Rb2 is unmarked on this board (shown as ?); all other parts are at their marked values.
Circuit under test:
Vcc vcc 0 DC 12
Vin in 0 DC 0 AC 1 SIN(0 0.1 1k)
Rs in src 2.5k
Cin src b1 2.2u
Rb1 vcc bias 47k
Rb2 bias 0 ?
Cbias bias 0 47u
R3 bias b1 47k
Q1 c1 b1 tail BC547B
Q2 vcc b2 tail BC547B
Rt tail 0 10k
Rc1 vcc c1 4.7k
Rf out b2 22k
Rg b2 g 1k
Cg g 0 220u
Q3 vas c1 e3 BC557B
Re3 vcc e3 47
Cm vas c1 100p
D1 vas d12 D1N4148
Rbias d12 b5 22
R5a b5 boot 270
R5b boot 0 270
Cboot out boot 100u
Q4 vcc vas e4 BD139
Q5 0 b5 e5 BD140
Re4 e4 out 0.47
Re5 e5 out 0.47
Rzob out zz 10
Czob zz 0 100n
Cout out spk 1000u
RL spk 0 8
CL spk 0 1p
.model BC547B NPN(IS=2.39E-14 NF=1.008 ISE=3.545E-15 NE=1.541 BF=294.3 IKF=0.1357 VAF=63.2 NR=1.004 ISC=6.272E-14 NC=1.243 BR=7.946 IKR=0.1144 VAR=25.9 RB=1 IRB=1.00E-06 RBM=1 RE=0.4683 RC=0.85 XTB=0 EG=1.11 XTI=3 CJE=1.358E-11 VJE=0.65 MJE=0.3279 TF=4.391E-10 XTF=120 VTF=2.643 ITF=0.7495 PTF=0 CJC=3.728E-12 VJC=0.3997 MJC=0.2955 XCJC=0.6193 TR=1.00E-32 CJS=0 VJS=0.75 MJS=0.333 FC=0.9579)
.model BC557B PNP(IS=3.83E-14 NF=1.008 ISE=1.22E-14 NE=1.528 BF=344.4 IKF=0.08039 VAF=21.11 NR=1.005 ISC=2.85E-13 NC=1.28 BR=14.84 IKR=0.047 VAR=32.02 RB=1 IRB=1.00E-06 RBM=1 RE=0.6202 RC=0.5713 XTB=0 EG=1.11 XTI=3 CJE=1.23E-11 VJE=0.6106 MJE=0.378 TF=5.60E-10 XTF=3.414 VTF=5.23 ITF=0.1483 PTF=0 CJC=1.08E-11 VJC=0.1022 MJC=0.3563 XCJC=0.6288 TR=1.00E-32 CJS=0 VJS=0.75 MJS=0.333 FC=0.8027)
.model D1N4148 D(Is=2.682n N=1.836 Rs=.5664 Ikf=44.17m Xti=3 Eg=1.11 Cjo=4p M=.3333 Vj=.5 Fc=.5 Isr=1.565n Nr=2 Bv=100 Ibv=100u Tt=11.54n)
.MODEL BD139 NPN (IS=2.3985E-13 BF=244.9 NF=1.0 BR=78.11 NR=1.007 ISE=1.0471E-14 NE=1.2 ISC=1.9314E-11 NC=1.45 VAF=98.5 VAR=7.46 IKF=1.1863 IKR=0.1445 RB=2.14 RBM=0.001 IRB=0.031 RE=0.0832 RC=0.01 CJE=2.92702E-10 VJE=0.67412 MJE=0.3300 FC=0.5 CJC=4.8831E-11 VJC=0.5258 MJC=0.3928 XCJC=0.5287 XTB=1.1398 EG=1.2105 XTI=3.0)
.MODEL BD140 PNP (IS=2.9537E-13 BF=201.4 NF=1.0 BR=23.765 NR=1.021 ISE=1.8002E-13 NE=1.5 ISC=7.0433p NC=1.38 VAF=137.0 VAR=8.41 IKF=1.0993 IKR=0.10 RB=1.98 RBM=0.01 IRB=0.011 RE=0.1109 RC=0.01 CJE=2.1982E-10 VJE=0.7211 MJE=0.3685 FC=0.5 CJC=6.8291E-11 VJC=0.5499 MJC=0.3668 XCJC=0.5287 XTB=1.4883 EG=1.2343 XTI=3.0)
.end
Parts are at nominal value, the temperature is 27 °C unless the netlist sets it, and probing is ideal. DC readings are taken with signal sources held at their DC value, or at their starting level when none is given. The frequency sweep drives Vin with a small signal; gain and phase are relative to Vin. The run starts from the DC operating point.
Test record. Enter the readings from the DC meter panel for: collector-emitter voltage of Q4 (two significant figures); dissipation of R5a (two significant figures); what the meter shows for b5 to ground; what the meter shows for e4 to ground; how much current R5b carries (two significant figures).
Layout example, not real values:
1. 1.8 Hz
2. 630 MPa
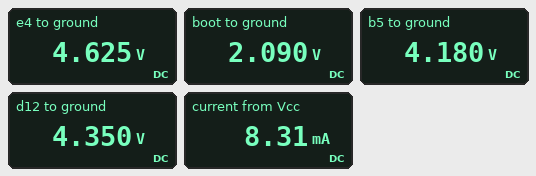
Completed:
1. 7.4 V
2. 16 mW
3. 4.180 V
4. 4.625 V
5. 7.7 mA
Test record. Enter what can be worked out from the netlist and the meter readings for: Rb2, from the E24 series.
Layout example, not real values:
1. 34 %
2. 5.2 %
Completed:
1. 30 kΩ
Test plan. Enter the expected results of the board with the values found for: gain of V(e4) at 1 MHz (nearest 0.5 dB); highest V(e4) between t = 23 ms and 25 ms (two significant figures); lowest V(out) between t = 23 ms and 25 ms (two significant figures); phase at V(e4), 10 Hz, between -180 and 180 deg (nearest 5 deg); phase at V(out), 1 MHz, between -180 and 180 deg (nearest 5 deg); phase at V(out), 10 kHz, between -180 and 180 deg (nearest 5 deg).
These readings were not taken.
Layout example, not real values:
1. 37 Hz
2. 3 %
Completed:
1. -20.5 dB
2. 6.7 V
3. 2.7 V
4. -20 deg
5. -80 deg
6. -10 deg
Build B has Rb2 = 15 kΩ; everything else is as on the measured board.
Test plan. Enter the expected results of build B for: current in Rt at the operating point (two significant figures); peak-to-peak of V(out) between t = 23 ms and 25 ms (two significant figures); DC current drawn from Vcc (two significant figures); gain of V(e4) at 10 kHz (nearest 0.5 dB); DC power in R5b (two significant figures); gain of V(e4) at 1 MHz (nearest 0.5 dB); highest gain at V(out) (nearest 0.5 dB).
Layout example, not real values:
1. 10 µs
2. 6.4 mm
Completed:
1. 230 µA
2. 2.9 V
3. 4.9 mA
4. -5.0 dB
5. 5.5 mW
6. -31.0 dB
7. 3.0 dB
